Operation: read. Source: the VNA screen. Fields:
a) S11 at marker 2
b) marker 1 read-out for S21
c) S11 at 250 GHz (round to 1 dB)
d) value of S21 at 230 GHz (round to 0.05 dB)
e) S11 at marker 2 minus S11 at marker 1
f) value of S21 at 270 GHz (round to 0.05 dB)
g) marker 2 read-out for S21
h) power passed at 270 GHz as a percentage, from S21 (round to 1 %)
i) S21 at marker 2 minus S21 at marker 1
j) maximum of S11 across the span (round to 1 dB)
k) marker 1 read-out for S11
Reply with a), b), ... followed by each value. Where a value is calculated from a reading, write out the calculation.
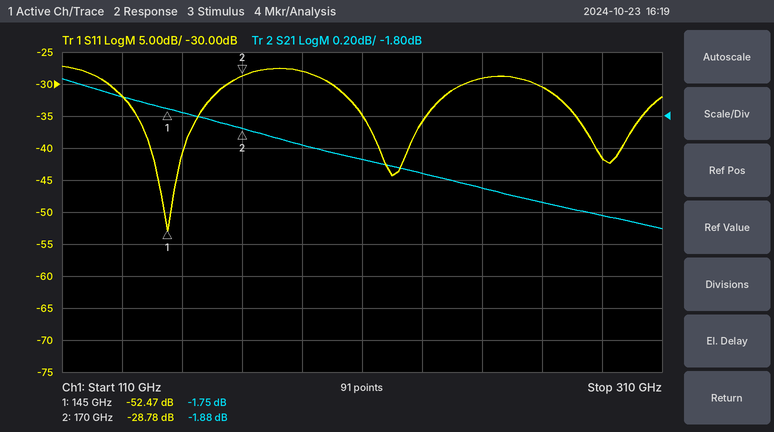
a) -28.78 dB
b) -1.75 dB
c) -29 dB
d) -2.15 dB
e) -28.78 − (-52.47) = 23.69 dB
f) -2.35 dB
g) -1.88 dB
h) 10^(-2.35/10) ≈ 58 %
i) -1.88 − (-1.75) = -0.13 dB
j) -27 dB
k) -52.47 dB
